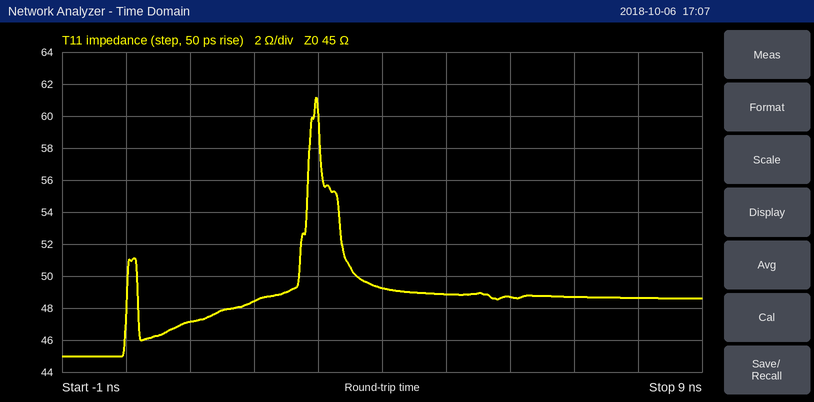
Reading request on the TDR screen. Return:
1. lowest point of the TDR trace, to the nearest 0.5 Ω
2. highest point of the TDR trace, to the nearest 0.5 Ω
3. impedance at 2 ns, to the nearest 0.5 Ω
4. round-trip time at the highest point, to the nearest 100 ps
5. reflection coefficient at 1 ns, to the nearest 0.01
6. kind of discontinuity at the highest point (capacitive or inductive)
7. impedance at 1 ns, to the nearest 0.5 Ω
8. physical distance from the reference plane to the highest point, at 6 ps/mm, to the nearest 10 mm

45.0 Ω
61.0 Ω
48.5 Ω
3.0 ns
+0.02
inductive
47.0 Ω
250 mm
